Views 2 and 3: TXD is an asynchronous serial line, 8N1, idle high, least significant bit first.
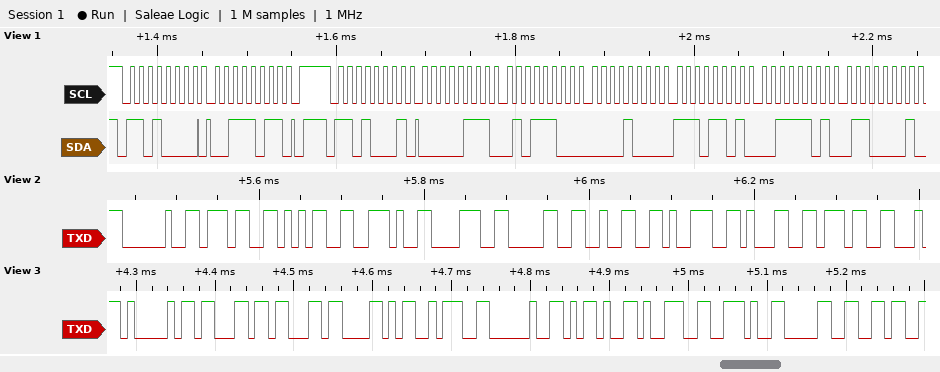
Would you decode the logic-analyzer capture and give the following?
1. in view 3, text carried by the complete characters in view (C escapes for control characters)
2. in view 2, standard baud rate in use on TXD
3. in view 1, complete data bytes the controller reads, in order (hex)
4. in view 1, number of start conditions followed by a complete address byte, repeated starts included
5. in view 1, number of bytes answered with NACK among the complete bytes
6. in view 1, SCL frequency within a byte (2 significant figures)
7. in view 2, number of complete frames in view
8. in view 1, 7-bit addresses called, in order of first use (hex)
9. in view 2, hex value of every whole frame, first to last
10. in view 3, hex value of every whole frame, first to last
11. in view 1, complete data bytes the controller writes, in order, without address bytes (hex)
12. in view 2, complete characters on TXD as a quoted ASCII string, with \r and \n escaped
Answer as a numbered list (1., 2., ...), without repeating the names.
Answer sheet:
1. "AccX: -9.06"
2. 115200 baud
3. 07 5C 08 ED 3D 61
4. 2
5. 0
6. 100 kHz
7. 10
8. 0x68
9. 20 37 35 2E 38 30 32 39 31 37
10. 41 63 63 58 3A 20 2D 39 2E 30 36
11. 3B
12. " 75.802917"
